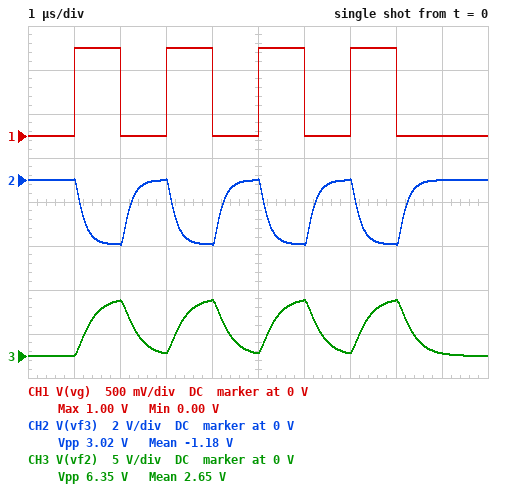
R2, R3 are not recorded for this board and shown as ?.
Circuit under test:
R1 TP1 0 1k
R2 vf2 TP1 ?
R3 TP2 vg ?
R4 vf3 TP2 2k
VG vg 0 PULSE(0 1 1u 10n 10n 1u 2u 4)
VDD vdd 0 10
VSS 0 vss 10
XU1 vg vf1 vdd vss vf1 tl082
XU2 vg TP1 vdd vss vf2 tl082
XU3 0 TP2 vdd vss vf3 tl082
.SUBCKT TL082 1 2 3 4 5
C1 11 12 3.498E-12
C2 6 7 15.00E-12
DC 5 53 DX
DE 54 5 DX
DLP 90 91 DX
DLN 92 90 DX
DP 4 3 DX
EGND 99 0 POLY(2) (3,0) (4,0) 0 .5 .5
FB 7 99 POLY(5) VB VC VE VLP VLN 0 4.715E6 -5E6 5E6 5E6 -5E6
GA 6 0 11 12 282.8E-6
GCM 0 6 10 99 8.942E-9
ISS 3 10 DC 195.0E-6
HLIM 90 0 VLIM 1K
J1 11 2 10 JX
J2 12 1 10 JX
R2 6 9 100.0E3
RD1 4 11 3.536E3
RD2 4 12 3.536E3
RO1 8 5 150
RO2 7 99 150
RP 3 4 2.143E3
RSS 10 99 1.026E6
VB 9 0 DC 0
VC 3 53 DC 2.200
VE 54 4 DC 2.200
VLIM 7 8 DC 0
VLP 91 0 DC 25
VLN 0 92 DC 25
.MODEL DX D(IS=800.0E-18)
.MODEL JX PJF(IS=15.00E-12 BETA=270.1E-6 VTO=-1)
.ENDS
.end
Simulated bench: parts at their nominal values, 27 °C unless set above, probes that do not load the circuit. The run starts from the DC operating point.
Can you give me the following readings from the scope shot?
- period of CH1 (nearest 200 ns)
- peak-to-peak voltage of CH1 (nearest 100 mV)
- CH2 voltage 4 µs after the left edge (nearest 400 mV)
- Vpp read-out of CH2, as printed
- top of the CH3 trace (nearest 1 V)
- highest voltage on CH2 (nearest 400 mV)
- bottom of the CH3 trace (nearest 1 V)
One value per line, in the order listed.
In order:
2.0 µs
1.0 V
-2.8 V
3.02 V
6 V
0 V
0 V
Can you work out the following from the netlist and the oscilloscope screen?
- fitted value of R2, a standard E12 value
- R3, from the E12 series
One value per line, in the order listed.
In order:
5.6 kΩ
680 Ω
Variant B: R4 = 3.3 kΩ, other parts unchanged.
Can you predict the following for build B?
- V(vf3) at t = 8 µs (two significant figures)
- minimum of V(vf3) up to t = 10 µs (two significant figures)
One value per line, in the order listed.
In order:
-4.7 V
-4.8 V
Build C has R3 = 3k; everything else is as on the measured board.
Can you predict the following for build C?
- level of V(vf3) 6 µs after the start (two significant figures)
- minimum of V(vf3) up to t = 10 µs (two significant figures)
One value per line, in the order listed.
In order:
-670 mV
-690 mV
